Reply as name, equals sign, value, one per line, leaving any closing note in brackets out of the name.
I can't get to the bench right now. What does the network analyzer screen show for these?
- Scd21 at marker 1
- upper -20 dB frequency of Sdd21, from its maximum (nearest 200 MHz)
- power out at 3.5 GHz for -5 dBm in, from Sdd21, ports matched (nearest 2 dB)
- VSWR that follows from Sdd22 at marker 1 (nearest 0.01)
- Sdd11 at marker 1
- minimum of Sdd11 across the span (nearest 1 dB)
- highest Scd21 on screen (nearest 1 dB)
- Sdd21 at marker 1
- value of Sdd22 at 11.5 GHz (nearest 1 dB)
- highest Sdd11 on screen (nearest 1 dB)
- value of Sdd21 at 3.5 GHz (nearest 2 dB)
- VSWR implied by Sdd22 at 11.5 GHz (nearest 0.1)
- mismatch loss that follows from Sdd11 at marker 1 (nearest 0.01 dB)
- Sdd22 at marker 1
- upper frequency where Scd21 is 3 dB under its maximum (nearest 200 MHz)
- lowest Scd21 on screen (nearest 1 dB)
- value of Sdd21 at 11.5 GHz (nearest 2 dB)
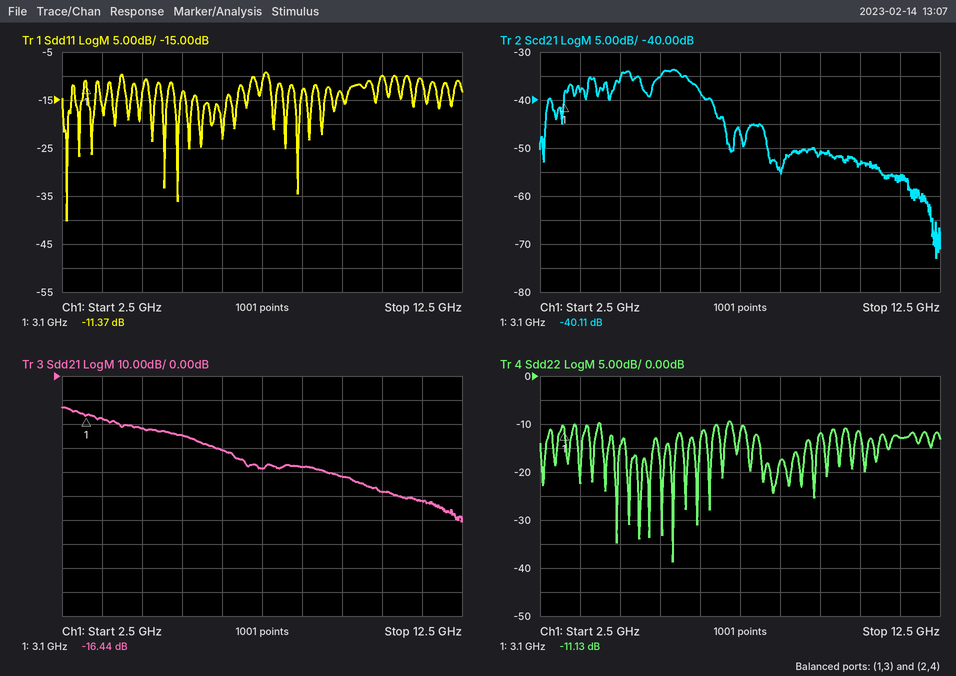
Scd21 at marker 1 = -40.11 dB
upper -20 dB frequency of Sdd21, from its maximum = 6.8 GHz
power out at 3.5 GHz for -5 dBm in, from Sdd21, ports matched = -22 dBm
VSWR that follows from Sdd22 at marker 1 = 1.77
Sdd11 at marker 1 = -11.37 dB
minimum of Sdd11 across the span = -40 dB
highest Scd21 on screen = -34 dB
Sdd21 at marker 1 = -16.44 dB
value of Sdd22 at 11.5 GHz = -13 dB
highest Sdd11 on screen = -9 dB
value of Sdd21 at 3.5 GHz = -18 dB
VSWR implied by Sdd22 at 11.5 GHz = 1.6
mismatch loss that follows from Sdd11 at marker 1 = 0.33 dB
Sdd22 at marker 1 = -11.13 dB
upper frequency where Scd21 is 3 dB under its maximum = 6.4 GHz
lowest Scd21 on screen = -73 dB
value of Sdd21 at 11.5 GHz = -52 dB
